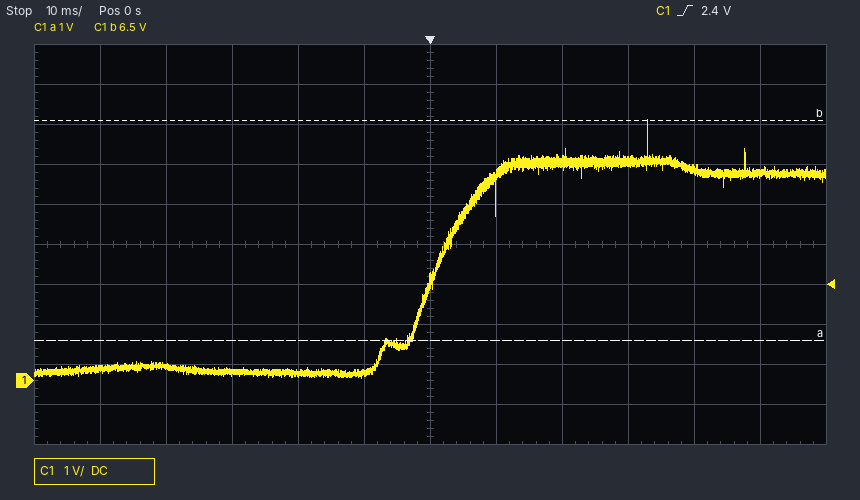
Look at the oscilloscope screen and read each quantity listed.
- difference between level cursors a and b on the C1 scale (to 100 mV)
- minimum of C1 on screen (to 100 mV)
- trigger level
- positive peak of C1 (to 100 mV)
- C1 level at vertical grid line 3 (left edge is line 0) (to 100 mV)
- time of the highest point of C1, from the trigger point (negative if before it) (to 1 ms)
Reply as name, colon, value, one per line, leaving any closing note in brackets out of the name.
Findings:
difference between level cursors a and b on the C1 scale: 5.5 V
minimum of C1 on screen: 100 mV
trigger level: 2.4 V
positive peak of C1: 6.5 V
C1 level at vertical grid line 3 (left edge is line 0): 200 mV
time of the highest point of C1, from the trigger point (negative if before it): +33 ms
